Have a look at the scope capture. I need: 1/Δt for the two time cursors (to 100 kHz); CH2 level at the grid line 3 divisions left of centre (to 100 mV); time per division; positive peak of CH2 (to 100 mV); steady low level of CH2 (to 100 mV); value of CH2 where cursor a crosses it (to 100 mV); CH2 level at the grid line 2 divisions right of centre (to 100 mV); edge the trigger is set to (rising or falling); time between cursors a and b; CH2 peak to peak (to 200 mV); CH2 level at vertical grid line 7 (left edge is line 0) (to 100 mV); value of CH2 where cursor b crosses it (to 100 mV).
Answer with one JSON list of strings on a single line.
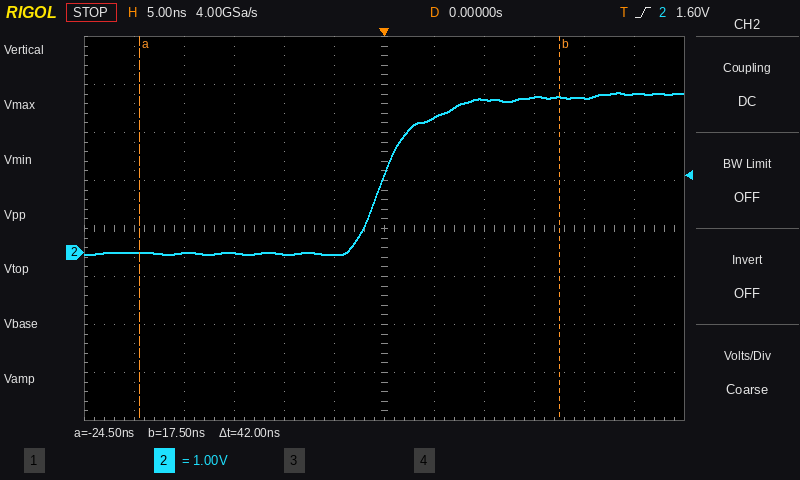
["23.8 MHz", "0.0 V", "5 ns", "3.3 V", "0.0 V", "0.0 V", "3.2 V", "rising", "42 ns", "3.4 V", "2.8 V", "3.2 V"]
